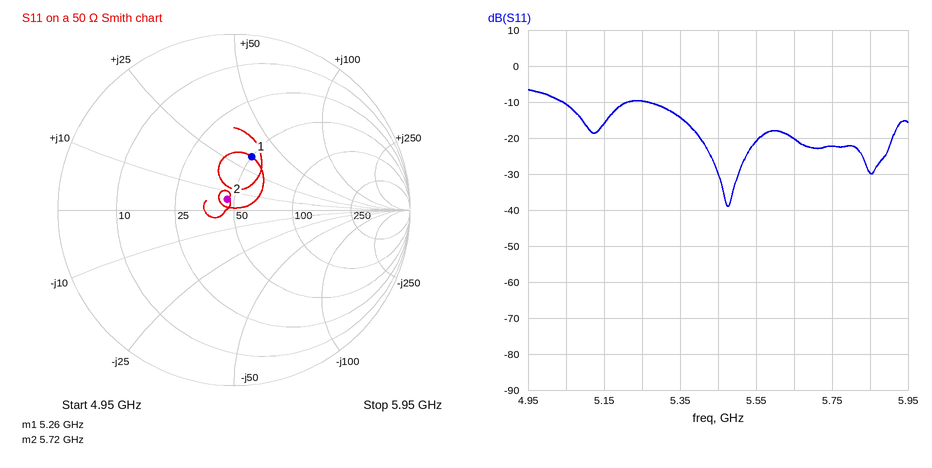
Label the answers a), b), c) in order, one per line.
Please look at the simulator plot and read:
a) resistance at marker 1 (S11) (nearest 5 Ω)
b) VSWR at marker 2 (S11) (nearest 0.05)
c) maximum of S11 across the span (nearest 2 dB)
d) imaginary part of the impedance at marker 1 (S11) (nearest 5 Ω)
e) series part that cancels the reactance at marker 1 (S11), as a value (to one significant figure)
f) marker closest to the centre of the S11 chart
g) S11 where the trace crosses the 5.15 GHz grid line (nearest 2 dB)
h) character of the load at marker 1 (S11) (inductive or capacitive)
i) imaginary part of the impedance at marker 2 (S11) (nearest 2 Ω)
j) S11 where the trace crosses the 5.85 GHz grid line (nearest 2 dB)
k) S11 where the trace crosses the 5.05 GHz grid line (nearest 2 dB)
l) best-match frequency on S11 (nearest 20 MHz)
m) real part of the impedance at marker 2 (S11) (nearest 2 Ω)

a) 50 Ω
b) 1.15
c) -6 dB
d) +35 Ω
e) 900 fF
f) marker 2
g) -16 dB
h) inductive
i) +6 Ω
j) -30 dB
k) -10 dB
l) 5.48 GHz
m) 46 Ω
